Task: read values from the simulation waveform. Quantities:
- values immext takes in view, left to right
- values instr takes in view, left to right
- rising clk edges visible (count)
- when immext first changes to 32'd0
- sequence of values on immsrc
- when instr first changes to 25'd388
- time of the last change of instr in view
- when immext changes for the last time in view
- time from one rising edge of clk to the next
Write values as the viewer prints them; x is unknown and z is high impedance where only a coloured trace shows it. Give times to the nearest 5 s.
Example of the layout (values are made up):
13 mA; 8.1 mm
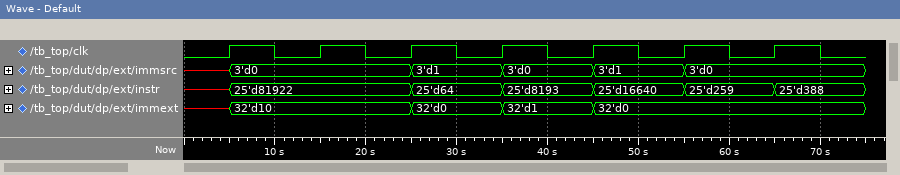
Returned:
x, 32'd10, 32'd0, 32'd1, 32'd0; x, 25'd81922, 25'd64, 25'd8193, 25'd16640, 25'd259, 25'd388; 7; 25 s; x, 3'd0, 3'd1, 3'd0, 3'd1, 3'd0; 65 s; 65 s; 45 s; 10 s
